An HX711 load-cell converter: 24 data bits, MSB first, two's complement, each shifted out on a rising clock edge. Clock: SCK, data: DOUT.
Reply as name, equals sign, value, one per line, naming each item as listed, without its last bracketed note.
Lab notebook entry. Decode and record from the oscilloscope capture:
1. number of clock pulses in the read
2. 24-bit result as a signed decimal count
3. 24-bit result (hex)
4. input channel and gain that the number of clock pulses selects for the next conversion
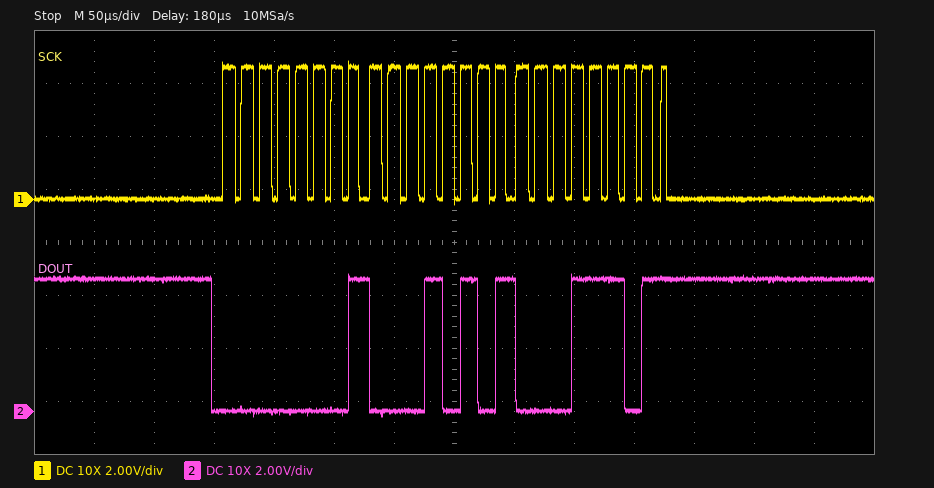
number of clock pulses in the read = 25
24-bit result as a signed decimal count = 70941
24-bit result = 0x01151D
input channel and gain that the number of clock pulses selects for the next conversion = channel A, gain 128
